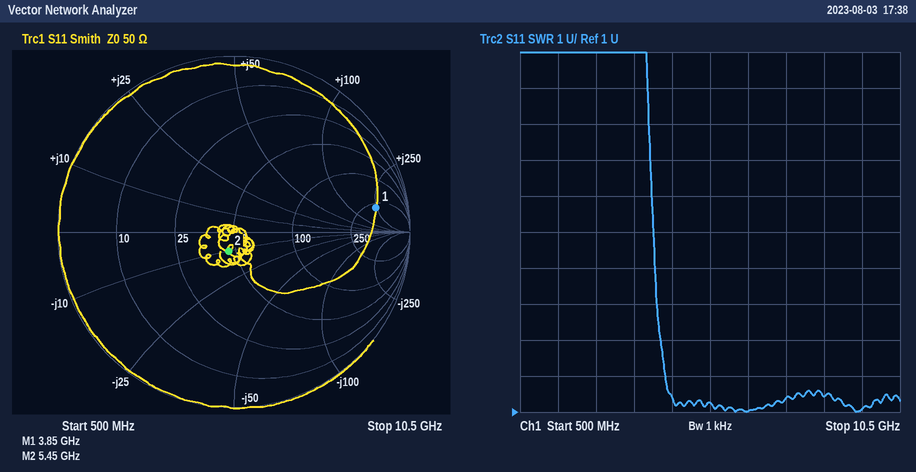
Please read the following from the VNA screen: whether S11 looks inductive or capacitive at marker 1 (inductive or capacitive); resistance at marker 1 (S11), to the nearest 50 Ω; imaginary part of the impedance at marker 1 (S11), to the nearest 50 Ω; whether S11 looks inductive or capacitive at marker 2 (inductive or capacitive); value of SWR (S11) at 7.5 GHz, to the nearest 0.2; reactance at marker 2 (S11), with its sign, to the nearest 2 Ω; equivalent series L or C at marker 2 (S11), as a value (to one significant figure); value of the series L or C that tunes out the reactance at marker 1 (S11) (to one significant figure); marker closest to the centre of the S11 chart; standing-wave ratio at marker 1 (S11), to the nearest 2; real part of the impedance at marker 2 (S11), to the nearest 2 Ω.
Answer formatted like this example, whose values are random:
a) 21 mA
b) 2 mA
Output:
a) inductive
b) 300 Ω
c) +250 Ω
d) capacitive
e) 1.4
f) -10 Ω
g) 3 pF
h) 200 fF
i) marker 2
j) 10
k) 46 Ω
